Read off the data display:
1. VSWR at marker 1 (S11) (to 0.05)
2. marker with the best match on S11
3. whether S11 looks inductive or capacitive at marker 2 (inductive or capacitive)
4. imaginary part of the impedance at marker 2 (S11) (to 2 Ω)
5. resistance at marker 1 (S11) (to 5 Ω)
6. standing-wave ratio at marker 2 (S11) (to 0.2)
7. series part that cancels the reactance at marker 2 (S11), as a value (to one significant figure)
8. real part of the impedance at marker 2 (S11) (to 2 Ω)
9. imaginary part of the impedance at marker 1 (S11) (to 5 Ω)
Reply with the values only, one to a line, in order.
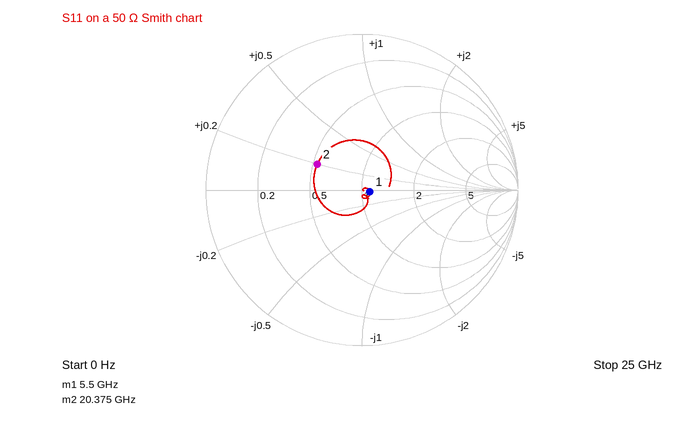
1.10
marker 1
inductive
+10 Ω
55 Ω
2.0
800 fF
26 Ω
0 Ω
